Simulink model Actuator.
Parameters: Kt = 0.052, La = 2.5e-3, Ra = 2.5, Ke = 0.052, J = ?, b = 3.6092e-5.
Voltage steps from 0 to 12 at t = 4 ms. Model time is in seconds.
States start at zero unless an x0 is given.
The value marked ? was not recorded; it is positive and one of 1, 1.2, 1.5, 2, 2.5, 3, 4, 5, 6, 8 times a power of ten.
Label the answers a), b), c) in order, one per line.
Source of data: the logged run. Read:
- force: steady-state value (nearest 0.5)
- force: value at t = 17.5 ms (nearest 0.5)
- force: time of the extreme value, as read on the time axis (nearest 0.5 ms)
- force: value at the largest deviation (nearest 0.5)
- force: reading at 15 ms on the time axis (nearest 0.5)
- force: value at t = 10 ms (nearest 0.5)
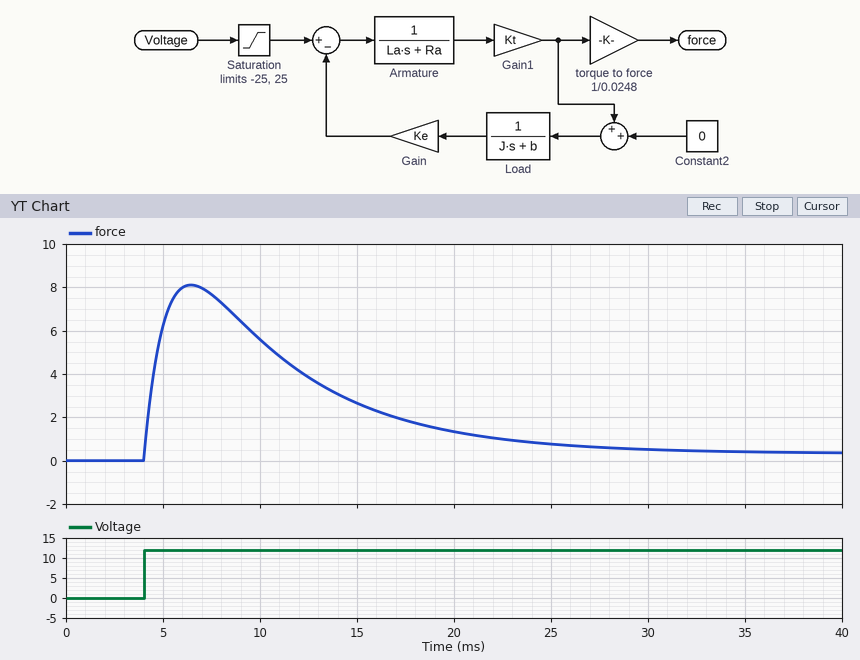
a) 0.5
b) 2.0
c) 6.5 ms
d) 8.0
e) 2.5
f) 5.5
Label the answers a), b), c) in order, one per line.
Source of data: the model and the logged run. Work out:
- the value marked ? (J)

a) 8e-06
